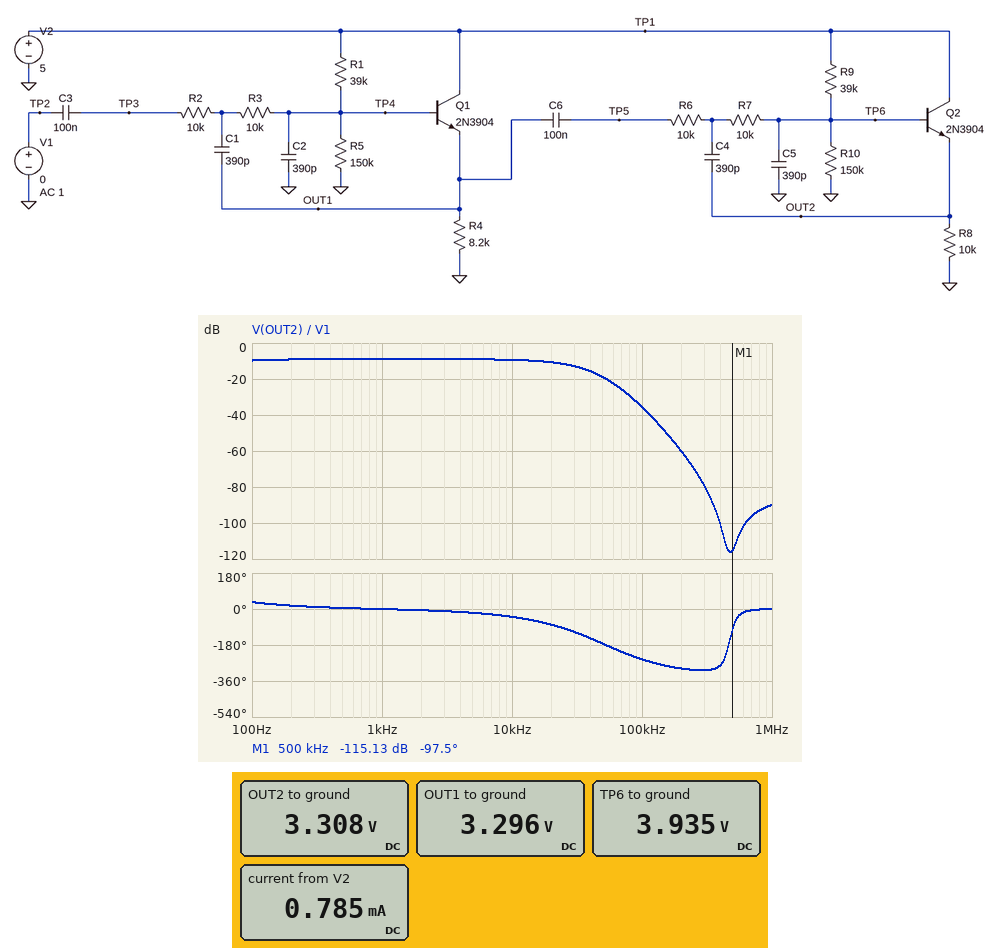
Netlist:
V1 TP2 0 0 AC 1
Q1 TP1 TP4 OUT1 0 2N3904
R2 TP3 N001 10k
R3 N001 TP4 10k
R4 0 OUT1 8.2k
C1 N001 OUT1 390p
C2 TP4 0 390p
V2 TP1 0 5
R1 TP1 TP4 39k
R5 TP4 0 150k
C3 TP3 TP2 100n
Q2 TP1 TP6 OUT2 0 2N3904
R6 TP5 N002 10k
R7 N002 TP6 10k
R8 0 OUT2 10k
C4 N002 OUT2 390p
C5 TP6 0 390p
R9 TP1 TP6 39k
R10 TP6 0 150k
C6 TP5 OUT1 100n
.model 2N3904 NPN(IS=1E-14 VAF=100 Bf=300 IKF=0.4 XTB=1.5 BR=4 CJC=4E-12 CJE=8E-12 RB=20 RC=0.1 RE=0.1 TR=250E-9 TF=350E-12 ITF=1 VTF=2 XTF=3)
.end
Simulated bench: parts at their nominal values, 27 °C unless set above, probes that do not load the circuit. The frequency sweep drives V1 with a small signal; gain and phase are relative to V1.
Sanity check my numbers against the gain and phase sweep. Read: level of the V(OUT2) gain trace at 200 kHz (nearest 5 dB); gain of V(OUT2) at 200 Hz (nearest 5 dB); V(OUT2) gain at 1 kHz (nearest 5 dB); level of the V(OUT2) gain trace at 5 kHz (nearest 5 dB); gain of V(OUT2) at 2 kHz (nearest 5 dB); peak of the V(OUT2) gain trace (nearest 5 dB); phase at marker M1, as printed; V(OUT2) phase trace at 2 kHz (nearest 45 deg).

-60 dB
-10 dB
-10 dB
-10 dB
-10 dB
-10 dB
-97.5 deg
0 deg
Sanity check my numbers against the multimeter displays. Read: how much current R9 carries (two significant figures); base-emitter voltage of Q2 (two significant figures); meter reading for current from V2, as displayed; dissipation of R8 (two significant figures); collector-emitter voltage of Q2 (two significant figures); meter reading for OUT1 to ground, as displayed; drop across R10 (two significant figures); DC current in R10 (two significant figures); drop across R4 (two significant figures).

27 µA
630 mV
0.785 mA
1.1 mW
1.7 V
3.296 V
3.9 V
26 µA
3.3 V
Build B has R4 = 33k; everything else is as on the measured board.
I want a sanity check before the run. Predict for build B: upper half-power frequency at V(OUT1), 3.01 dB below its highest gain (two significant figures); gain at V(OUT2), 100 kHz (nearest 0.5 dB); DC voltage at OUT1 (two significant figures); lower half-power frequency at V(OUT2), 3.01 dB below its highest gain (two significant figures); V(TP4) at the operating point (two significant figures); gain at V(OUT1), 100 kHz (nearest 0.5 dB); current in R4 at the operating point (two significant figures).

36 kHz
-37.0 dB
3.4 V
48 Hz
4.0 V
-19.5 dB
100 µA
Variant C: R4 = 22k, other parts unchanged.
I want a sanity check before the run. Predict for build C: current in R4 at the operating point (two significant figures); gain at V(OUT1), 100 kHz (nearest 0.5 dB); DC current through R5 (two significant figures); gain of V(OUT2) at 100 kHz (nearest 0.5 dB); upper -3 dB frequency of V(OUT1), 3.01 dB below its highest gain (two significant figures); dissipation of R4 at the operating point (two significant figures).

150 µA
-18.5 dB
26 µA
-36.5 dB
37 kHz
510 µW
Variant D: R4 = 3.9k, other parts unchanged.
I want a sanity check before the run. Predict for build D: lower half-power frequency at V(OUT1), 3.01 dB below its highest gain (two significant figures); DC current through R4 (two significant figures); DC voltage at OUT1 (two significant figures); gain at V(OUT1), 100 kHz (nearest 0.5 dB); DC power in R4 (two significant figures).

32 Hz
830 µA
3.2 V
-17.5 dB
2.7 mW
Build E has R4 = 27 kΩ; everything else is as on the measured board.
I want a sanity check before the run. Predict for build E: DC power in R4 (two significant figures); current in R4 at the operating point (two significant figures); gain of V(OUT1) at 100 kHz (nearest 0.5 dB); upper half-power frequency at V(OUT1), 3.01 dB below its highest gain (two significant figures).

420 µW
120 µA
-19.0 dB
36 kHz
